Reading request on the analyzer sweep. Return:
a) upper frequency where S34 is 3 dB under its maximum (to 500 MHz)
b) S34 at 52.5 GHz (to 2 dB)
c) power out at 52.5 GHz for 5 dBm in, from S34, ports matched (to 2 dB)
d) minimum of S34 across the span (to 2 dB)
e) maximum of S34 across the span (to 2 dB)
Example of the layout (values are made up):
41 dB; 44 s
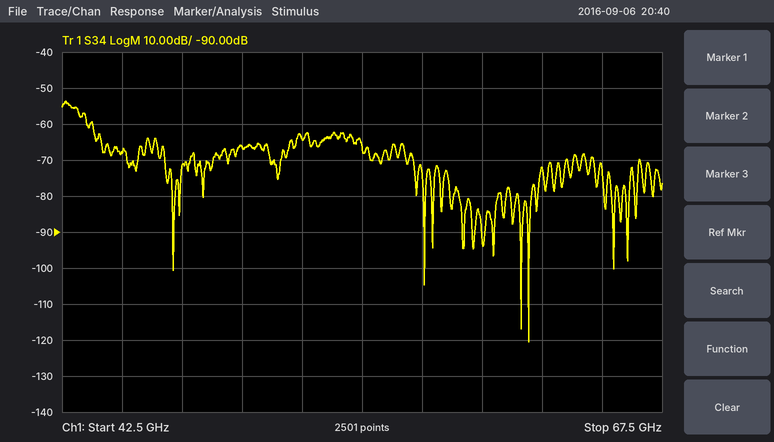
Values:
43.0 GHz; -64 dB; -60 dBm; -120 dB; -54 dB
